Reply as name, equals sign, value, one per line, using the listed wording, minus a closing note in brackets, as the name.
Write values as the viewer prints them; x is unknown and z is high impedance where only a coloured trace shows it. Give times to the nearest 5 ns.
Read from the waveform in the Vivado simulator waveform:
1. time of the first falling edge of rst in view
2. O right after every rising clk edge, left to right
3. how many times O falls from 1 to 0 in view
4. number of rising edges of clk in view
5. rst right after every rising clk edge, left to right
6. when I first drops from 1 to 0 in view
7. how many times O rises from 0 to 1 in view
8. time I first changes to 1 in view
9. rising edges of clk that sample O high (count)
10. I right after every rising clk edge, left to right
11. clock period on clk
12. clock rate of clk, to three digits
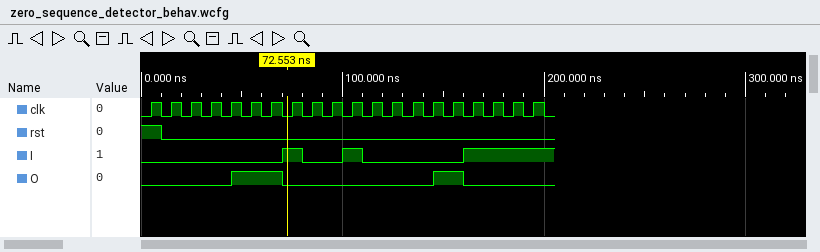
time of the first falling edge of rst in view = 10 ns
O right after every rising clk edge, left to right = 0 0 0 0 1 1 1 0 0 0 0 0 0 0 1 1 0 0 0 0
how many times O falls from 1 to 0 in view = 2
number of rising edges of clk in view = 20
rst right after every rising clk edge, left to right = 1 0 0 0 0 0 0 0 0 0 0 0 0 0 0 0 0 0 0 0
when I first drops from 1 to 0 in view = 80 ns
how many times O rises from 0 to 1 in view = 2
time I first changes to 1 in view = 70 ns
rising edges of clk that sample O high = 3
I right after every rising clk edge, left to right = 0 0 0 0 0 0 0 1 0 0 1 0 0 0 0 0 1 1 1 1
clock period on clk = 10 ns
clock rate of clk, to three digits = 100 MHz
